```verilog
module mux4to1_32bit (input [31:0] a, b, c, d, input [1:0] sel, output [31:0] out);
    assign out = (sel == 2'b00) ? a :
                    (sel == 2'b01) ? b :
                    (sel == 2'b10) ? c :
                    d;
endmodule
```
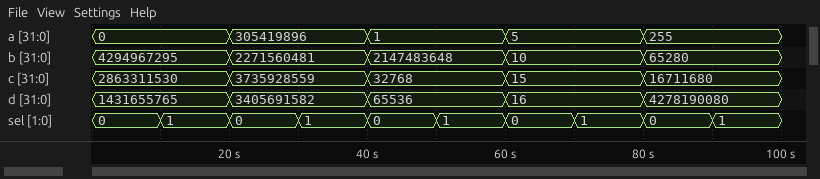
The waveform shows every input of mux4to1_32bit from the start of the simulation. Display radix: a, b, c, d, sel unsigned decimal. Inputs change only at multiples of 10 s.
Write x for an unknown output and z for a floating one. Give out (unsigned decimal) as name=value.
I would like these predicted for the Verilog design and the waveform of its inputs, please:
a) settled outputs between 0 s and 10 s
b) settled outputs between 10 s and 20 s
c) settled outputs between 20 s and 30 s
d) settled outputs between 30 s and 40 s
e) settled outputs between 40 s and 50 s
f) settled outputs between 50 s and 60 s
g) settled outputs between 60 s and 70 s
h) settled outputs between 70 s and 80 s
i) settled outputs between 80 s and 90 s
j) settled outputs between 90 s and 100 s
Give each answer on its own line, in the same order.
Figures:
out=0
out=4294967295
out=305419896
out=2271560481
out=1
out=2147483648
out=5
out=10
out=255
out=65280
